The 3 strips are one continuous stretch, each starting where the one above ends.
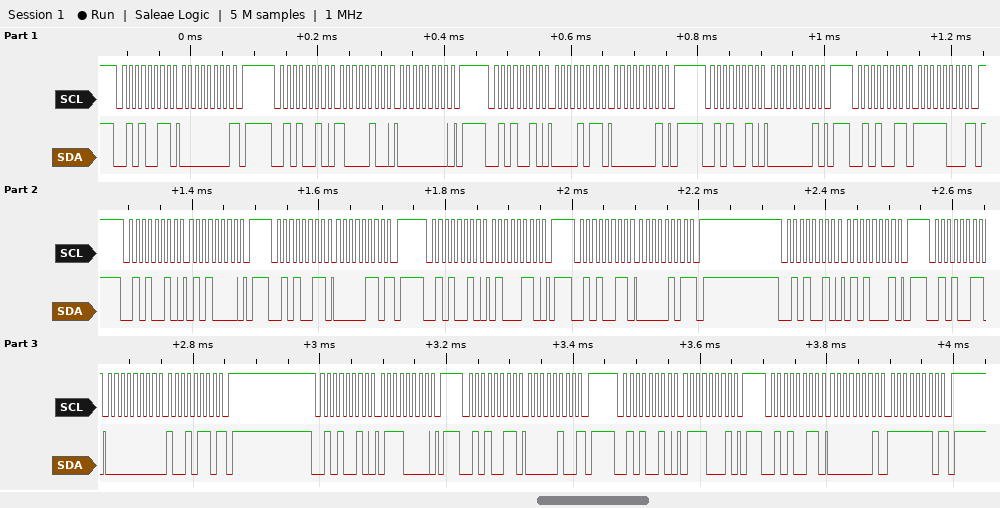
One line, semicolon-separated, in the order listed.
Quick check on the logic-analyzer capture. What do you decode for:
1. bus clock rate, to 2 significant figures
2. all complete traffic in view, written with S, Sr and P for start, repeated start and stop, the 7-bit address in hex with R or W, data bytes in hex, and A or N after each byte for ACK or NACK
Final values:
100 kHz; S 29R A 00 N P S 29W A 84 A 00 A P S 29W A 0B A 01 A P S 29W A 01 A P S 29R A F8 N P S 29W A 50 A P S 29R A 06 N P S 29W A 46 A P S 29R A 05 N P S 29W A 51 A P S 29R A 00 A 96 N P S 29W A 70 A P S 29R A 04 N P S 29W A 71 A P S 29R A 01 A FE N P
